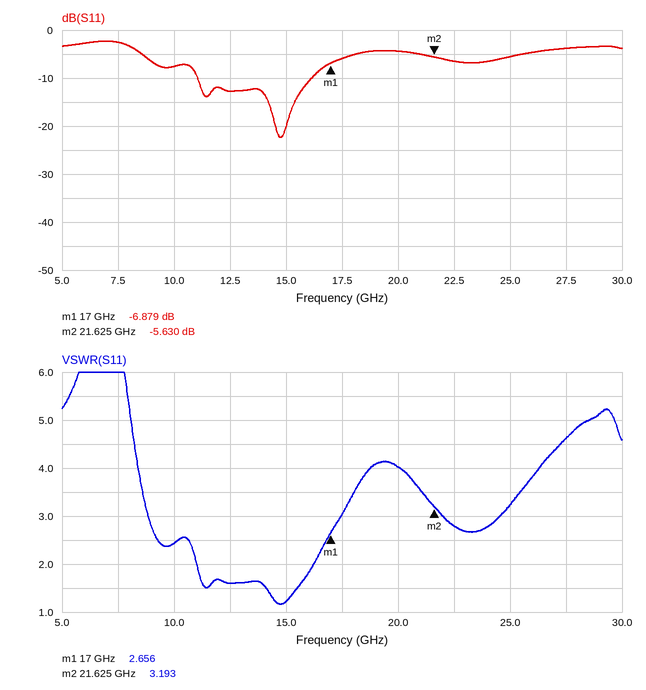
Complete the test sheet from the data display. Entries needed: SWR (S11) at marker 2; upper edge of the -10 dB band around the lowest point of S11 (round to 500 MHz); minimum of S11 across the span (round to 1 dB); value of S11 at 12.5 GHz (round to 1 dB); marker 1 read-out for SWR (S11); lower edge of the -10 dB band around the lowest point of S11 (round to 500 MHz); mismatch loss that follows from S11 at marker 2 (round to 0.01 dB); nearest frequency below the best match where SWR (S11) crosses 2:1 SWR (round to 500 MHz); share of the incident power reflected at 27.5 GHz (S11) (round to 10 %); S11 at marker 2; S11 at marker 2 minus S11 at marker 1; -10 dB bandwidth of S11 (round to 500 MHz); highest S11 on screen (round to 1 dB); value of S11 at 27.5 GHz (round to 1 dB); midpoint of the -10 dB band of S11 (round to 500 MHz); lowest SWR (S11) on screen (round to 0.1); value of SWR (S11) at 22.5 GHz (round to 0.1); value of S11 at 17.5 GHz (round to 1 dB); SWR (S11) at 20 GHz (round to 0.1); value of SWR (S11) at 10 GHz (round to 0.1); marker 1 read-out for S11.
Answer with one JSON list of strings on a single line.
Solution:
["3.193", "16.0 GHz", "-22 dB", "-13 dB", "2.656", "11.0 GHz", "1.39 dB", "11.0 GHz", "40 %", "-5.630 dB", "1.249 dB", "5.0 GHz", "-2 dB", "-4 dB", "13.5 GHz", "1.2", "2.8", "-6 dB", "4.0", "2.4", "-6.879 dB"]
